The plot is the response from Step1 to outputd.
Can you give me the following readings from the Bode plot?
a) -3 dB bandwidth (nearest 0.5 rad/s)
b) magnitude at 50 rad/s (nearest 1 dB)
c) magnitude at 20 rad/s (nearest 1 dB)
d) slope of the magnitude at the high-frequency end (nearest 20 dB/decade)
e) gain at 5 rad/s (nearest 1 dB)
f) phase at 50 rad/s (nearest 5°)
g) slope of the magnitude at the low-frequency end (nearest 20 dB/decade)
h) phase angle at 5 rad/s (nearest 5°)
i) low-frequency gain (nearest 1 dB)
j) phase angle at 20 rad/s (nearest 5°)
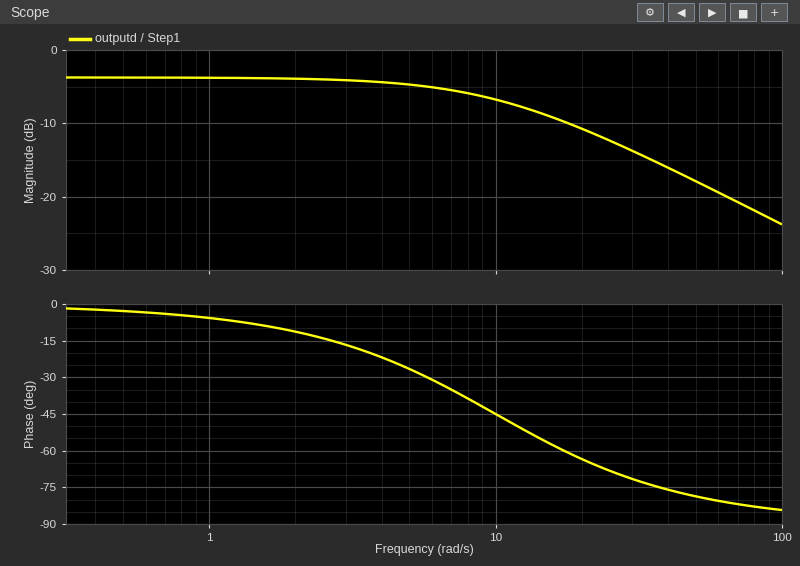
10.0 rad/s
-18 dB
-11 dB
-20 dB/decade
-5 dB
-80°
0 dB/decade
-25°
-4 dB
-65°
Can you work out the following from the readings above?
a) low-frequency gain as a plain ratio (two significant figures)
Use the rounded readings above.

0.63
